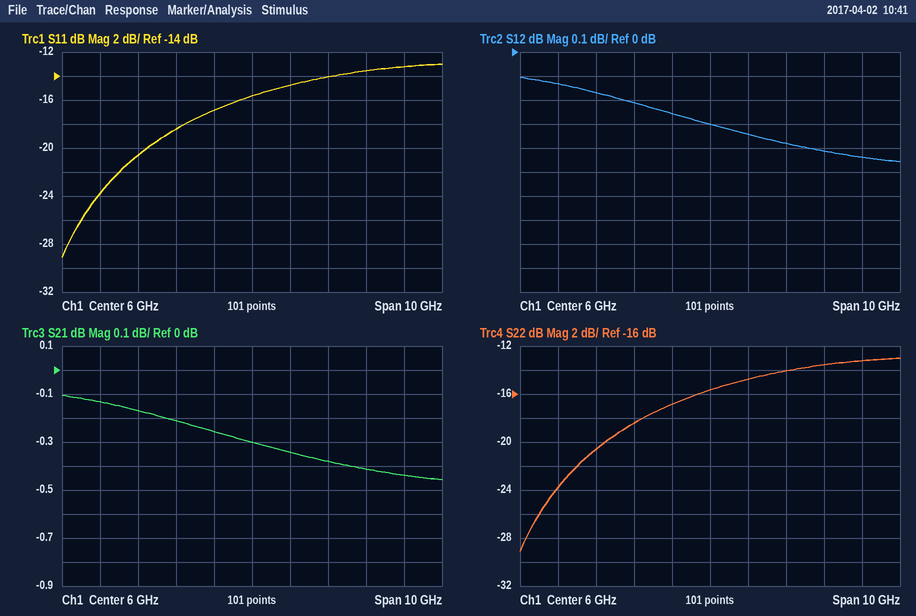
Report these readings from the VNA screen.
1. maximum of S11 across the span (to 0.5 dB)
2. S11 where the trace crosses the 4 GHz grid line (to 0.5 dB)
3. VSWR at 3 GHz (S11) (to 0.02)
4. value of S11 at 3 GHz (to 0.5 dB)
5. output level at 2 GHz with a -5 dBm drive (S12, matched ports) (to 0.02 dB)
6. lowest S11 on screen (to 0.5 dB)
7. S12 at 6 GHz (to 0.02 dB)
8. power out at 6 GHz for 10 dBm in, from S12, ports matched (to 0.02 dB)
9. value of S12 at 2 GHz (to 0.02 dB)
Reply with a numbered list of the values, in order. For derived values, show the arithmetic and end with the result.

1. -13.0 dB
2. -18.5 dB
3. |Γ| = 10^(-20.5/20) = 0.0944; VSWR = (1 + 0.0944)/(1 − 0.0944) ≈ 1.21, so 1.20 to the nearest 0.02
4. -20.5 dB
5. -5 dBm + (-0.14 dB) = -5.14 dBm
6. -29.0 dB
7. -0.30 dB
8. 10 dBm + (-0.30 dB) = 9.70 dBm
9. -0.14 dB
